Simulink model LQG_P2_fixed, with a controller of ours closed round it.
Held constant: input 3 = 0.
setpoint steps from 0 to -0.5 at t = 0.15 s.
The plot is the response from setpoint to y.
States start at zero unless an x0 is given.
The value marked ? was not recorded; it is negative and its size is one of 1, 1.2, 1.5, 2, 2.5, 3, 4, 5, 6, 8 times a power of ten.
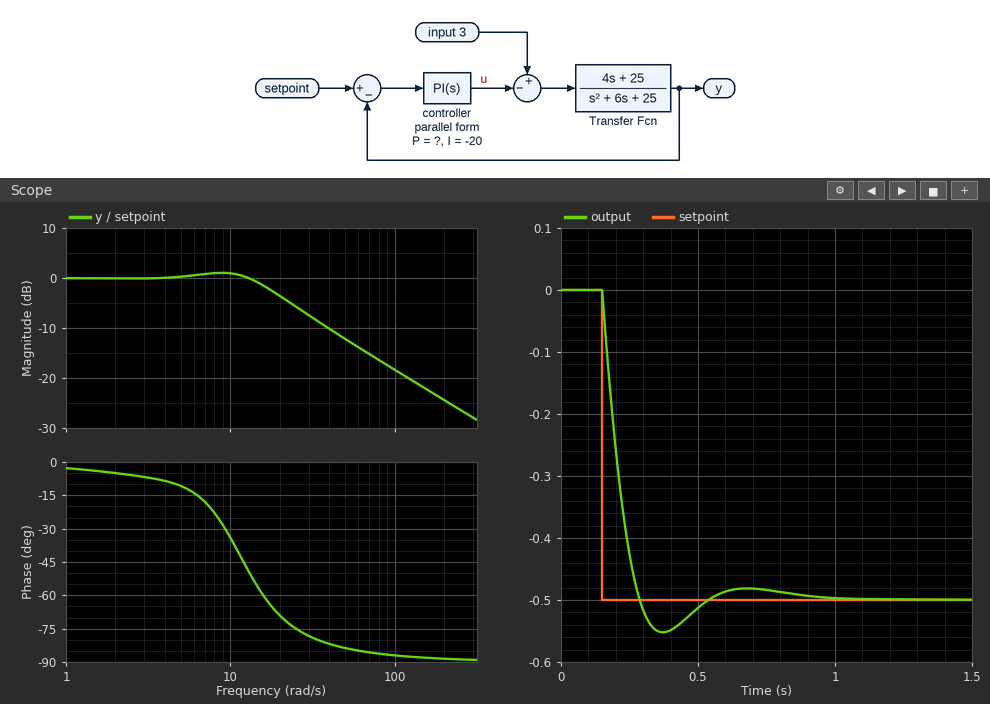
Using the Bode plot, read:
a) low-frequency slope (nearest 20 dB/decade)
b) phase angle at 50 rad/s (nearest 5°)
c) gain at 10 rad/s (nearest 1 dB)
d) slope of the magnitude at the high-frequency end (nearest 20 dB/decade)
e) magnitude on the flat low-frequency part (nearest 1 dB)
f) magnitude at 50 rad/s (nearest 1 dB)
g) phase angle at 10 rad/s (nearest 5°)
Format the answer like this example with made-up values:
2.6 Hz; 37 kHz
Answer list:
0 dB/decade; -85°; 1 dB; -20 dB/decade; 0 dB; -12 dB; -35°
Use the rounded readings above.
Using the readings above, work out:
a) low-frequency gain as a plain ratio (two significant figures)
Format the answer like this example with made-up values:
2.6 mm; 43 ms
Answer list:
1.0
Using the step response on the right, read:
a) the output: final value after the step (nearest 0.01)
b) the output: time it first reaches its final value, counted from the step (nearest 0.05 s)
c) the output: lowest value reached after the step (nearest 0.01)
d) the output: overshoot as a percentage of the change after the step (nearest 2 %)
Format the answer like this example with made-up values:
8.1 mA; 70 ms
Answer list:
-0.50; 0.15 s; -0.55; 10 %
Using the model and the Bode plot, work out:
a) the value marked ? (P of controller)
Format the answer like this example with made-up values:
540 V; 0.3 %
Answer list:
-3
